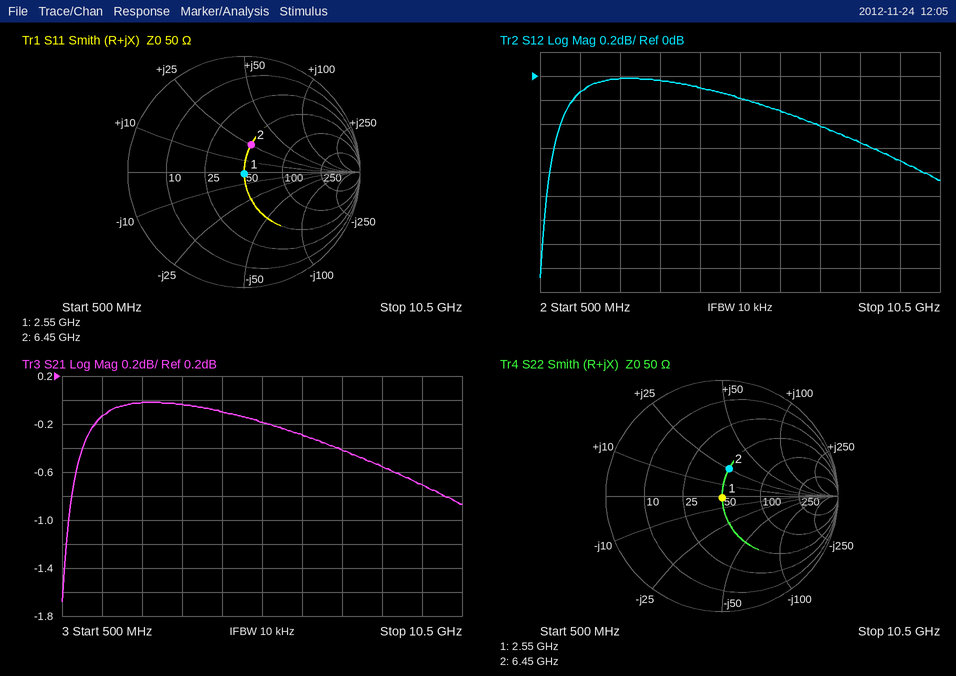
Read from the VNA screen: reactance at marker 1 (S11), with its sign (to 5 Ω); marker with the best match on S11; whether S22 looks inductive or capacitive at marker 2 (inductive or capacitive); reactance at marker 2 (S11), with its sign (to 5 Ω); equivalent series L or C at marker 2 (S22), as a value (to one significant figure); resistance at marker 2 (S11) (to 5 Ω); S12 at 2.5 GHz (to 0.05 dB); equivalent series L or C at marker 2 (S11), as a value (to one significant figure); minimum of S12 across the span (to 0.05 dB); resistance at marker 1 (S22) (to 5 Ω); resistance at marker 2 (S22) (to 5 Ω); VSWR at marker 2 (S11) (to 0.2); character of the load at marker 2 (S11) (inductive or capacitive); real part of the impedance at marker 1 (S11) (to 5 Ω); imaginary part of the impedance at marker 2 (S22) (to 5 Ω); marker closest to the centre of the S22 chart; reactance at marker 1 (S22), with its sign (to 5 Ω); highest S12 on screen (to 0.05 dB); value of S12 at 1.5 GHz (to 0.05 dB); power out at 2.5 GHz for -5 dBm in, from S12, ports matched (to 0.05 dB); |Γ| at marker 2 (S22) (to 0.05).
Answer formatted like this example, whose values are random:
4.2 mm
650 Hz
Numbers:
0 Ω
marker 1
inductive
+25 Ω
600 pH
50 Ω
0.00 dB
600 pH
-1.70 dB
50 Ω
50 Ω
1.6
inductive
50 Ω
+25 Ω
marker 1
0 Ω
0.00 dB
-0.15 dB
-5.00 dBm
0.25
